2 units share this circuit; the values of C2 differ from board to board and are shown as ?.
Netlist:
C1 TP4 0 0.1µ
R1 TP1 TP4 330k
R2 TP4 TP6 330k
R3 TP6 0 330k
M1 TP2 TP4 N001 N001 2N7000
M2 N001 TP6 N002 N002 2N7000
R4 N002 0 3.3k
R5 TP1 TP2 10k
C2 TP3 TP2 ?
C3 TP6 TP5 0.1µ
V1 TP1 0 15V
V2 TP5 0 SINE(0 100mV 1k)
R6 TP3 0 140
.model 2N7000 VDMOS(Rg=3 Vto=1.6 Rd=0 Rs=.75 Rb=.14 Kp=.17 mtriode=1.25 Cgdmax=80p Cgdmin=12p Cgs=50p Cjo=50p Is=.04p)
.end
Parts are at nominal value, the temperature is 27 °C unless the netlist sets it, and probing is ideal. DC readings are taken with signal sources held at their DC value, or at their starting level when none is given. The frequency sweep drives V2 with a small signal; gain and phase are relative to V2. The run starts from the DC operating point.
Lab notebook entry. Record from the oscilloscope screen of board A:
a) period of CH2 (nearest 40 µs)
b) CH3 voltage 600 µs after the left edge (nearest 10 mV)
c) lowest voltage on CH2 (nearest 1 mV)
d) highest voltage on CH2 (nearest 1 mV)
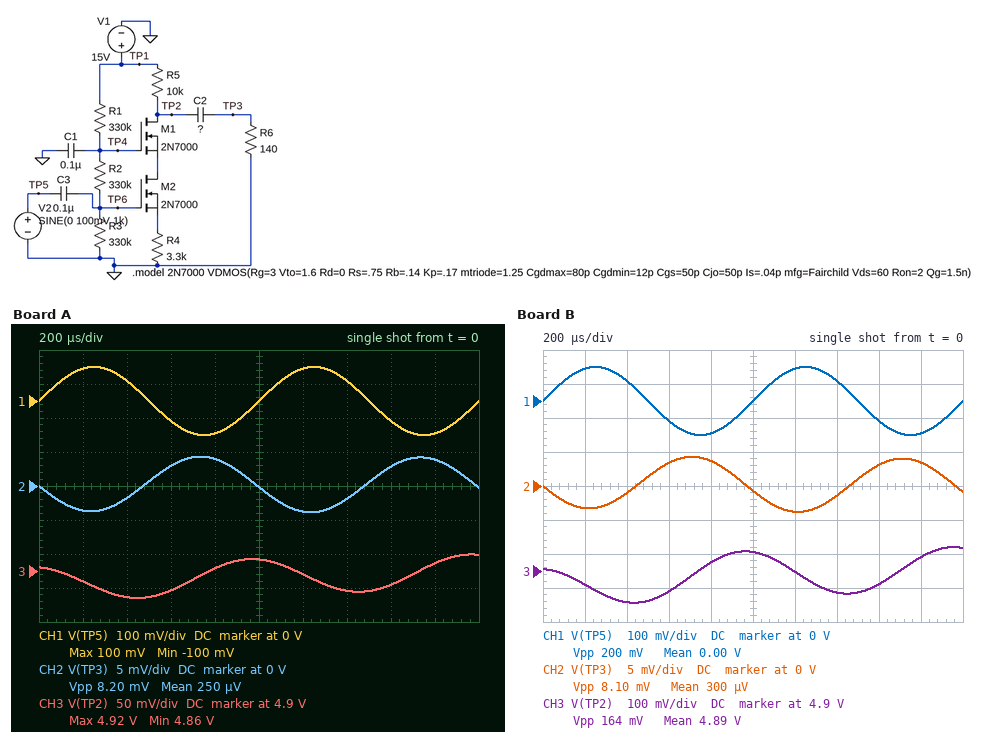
1.00 ms
4.87 V
-4 mV
4 mV
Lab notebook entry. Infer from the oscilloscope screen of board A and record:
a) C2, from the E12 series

180 nF
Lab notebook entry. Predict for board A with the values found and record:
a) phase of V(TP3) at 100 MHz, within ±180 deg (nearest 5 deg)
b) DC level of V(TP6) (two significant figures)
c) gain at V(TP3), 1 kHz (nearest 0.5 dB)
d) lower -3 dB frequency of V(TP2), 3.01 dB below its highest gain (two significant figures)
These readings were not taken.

5 deg
5.0 V
-28.0 dB
7.4 Hz
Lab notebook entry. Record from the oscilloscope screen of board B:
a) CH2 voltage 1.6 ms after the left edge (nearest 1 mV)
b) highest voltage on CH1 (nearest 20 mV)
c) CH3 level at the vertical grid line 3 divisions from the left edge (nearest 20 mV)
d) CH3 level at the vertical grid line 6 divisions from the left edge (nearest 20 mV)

3 mV
100 mV
4.84 V
4.90 V
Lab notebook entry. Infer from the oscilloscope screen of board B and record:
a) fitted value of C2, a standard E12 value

68 nF
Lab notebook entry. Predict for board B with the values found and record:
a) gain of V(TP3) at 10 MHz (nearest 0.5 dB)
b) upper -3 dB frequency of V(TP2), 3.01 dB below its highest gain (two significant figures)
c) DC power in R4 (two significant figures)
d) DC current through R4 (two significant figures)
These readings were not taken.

-11.0 dB
250 Hz
3.4 mW
1.0 mA
